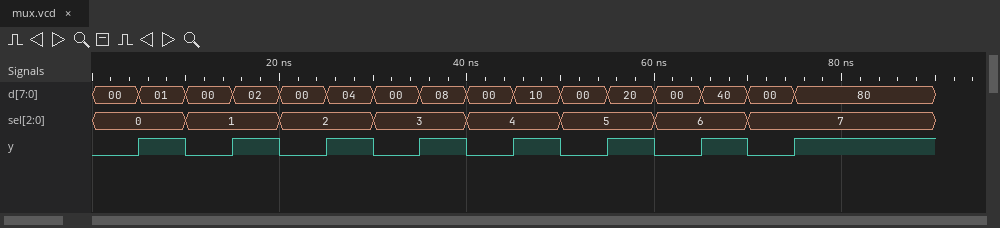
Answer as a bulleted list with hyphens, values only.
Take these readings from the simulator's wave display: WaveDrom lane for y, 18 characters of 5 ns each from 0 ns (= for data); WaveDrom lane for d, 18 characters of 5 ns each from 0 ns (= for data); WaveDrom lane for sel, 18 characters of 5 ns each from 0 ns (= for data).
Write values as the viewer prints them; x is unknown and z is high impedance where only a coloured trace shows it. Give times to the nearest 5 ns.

- {name: 'y', wave: '0101010101010101..'}
- {name: 'd', wave: '================..', data: '00 01 00 02 00 04 00 08 00 10 00 20 00 40 00 80'}
- {name: 'sel', wave: '=.=.=.=.=.=.=.=...', data: '0 1 2 3 4 5 6 7'}
